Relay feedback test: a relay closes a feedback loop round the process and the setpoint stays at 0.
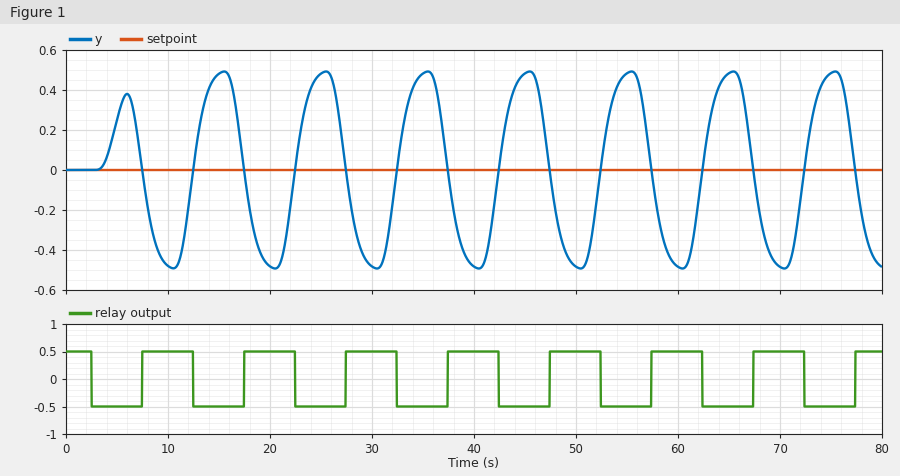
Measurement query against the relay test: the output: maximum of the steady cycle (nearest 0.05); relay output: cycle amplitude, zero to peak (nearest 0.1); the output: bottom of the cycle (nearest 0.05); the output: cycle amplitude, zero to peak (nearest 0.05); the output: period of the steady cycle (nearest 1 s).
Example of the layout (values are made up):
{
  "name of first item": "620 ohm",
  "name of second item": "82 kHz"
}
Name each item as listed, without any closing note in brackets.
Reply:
{
  "the output: maximum of the steady cycle": "0.50",
  "relay output: cycle amplitude, zero to peak": "0.5",
  "the output: bottom of the cycle": "-0.50",
  "the output: cycle amplitude, zero to peak": "0.50",
  "the output: period of the steady cycle": "10 s"
}
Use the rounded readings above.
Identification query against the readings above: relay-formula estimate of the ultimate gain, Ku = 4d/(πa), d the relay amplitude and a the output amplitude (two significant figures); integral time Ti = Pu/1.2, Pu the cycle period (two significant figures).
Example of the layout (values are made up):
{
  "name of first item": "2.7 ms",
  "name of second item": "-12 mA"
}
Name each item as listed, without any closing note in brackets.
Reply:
{
  "relay-formula estimate of the ultimate gain, Ku = 4d/(πa), d the relay amplitude and a the output amplitude": "1.3",
  "integral time Ti = Pu/1.2, Pu the cycle period": "8.3 s"
}
